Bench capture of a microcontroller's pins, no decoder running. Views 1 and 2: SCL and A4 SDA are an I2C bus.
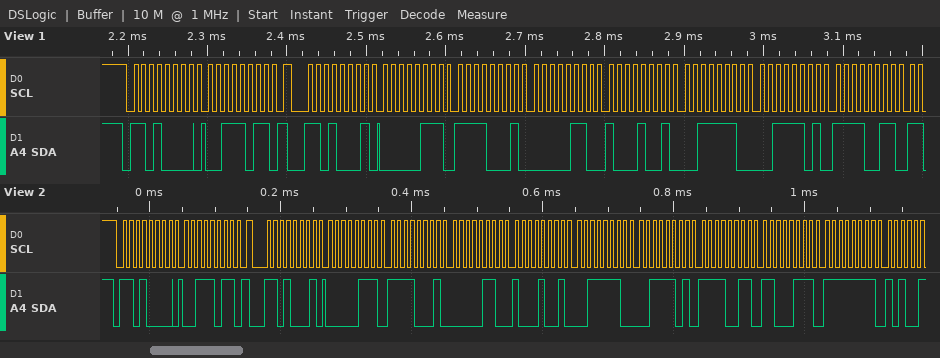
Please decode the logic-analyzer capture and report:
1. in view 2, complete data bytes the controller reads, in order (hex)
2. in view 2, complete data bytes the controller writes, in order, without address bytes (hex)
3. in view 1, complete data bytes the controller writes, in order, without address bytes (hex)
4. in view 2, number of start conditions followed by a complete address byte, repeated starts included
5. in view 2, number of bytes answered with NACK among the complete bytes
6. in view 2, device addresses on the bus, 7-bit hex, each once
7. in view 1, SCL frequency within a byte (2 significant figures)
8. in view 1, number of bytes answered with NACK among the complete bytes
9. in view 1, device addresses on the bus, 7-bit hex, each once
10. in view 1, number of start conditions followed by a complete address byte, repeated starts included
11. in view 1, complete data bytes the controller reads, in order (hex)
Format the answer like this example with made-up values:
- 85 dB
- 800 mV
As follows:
- 07 F1 06 89 3E 3D F3 C7 FF
- 3B
- 3B
- 2
- 0
- 0x68
- 100 kHz
- 0
- 0x68
- 2
- 07 F1 06 89 3E 3D F3
